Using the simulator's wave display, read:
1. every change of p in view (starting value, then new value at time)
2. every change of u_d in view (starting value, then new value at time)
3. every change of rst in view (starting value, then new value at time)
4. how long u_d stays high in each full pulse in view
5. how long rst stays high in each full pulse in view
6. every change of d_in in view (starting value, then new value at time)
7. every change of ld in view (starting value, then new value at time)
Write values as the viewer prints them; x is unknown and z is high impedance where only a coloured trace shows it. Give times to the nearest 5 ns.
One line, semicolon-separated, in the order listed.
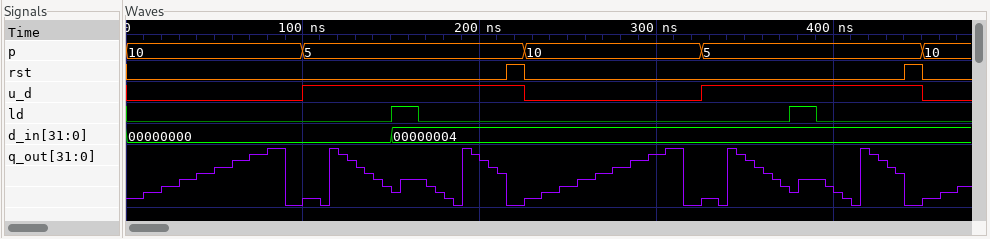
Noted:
10, 5 at 100 ns, 10 at 225 ns, 5 at 325 ns, 10 at 450 ns; 0, 1 at 100 ns, 0 at 225 ns, 1 at 325 ns, 0 at 450 ns; 0, 1 at 215 ns, 0 at 225 ns, 1 at 440 ns, 0 at 450 ns; 125 ns, 125 ns; 10 ns, 10 ns; 00000000, 00000004 at 150 ns; 0, 1 at 150 ns, 0 at 165 ns, 1 at 375 ns, 0 at 390 ns
